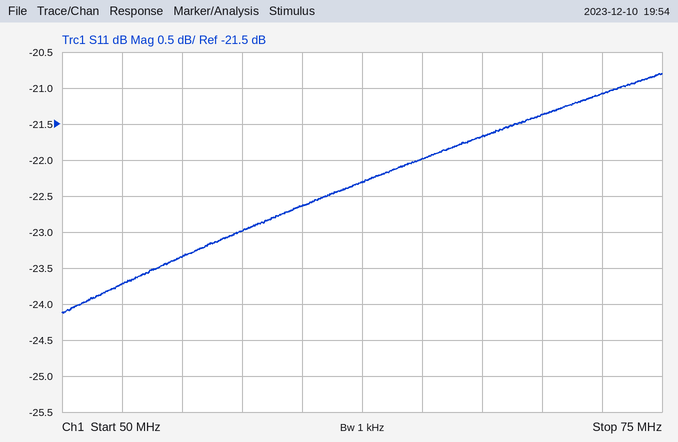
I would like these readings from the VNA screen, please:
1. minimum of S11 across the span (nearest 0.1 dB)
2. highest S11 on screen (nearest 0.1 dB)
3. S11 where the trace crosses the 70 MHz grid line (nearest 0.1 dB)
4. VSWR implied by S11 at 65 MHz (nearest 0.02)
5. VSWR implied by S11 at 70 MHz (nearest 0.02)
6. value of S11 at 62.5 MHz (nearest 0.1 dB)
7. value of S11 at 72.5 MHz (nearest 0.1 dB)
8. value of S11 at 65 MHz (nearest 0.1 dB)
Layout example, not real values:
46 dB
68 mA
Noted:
-24.1 dB
-20.8 dB
-21.4 dB
1.18
1.18
-22.3 dB
-21.1 dB
-22.0 dB
